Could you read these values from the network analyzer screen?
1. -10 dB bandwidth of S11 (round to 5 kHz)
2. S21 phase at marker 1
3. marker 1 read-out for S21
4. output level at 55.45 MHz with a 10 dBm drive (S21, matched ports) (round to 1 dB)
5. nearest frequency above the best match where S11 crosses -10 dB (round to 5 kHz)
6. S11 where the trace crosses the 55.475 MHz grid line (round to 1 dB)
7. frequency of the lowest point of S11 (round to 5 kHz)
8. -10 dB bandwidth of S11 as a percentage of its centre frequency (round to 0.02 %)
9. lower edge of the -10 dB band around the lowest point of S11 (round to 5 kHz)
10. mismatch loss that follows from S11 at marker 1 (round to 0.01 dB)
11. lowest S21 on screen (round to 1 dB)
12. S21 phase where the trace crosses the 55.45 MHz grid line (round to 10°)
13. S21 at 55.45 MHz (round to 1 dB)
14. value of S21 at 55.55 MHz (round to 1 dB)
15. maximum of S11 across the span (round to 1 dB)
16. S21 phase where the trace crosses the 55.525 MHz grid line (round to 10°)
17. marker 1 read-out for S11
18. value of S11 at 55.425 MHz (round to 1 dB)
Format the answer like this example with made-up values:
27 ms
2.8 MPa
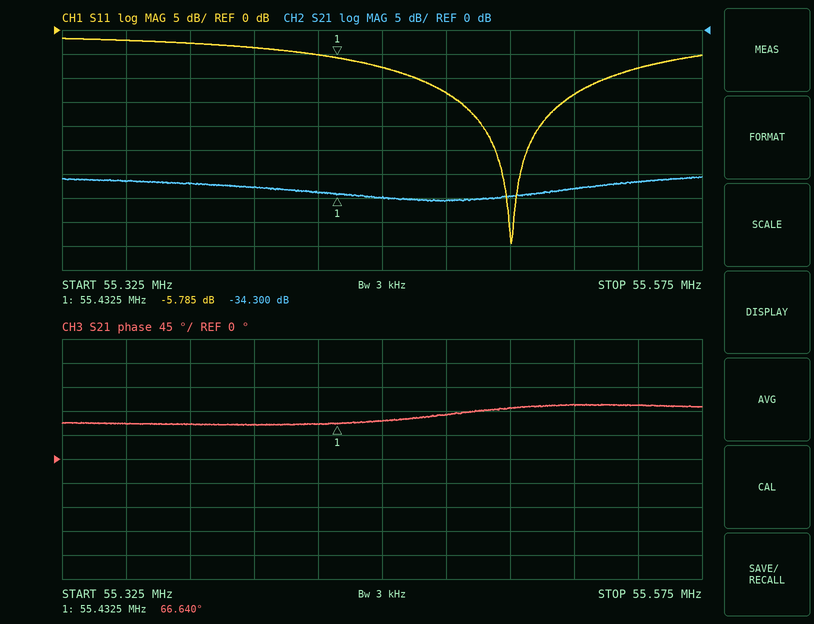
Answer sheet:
75 kHz
66.640°
-34.300 dB
-25 dBm
55.540 MHz
-13 dB
55.500 MHz
0.14 %
55.465 MHz
1.33 dB
-36 dB
70°
-35 dB
-32 dB
-2 dB
100°
-5.785 dB
-5 dB
